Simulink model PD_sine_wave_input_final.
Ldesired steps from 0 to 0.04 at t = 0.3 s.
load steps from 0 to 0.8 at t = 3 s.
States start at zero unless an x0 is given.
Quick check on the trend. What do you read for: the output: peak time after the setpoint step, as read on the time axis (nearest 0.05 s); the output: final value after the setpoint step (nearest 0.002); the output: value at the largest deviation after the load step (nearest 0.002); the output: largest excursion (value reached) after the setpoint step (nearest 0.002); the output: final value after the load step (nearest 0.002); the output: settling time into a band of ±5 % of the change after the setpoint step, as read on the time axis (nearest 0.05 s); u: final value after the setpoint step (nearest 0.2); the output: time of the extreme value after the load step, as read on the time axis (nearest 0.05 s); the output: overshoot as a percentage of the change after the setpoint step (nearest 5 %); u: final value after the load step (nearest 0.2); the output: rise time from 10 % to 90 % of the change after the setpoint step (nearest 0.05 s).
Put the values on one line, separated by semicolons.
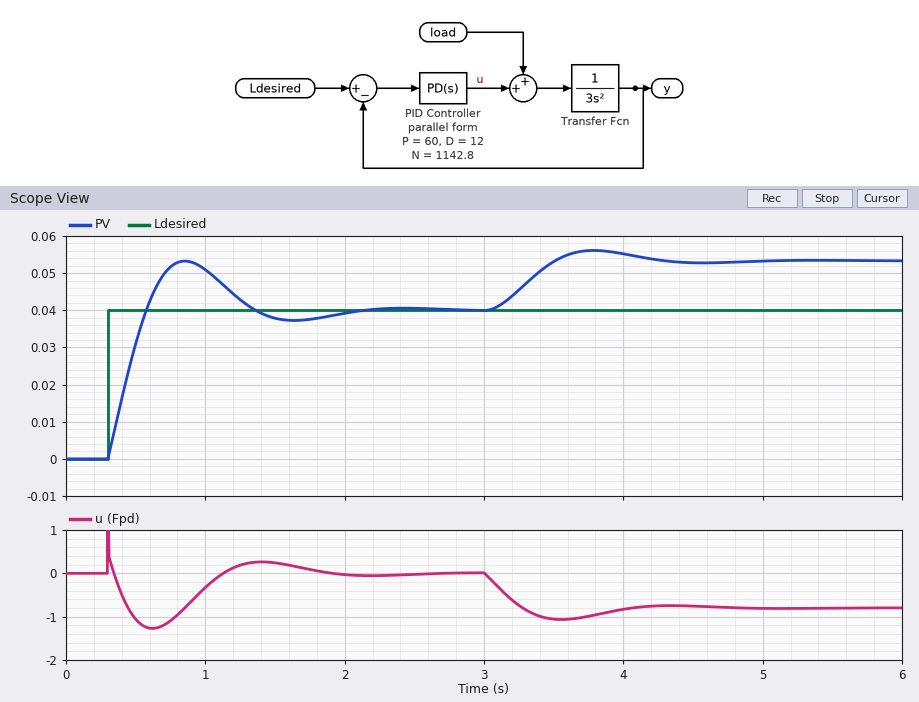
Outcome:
0.85 s; 0.040; 0.056; 0.054; 0.054; 1.85 s; 0.0; 3.80 s; 35 %; -0.8; 0.20 s
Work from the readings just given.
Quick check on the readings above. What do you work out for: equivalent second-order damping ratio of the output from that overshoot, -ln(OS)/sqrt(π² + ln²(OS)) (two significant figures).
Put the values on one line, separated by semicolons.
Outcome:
0.32
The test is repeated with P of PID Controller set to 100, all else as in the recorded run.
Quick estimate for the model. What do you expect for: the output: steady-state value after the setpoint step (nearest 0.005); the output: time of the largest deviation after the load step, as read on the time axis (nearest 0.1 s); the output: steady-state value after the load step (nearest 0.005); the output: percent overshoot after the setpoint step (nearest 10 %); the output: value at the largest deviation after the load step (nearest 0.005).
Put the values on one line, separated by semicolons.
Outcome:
0.040; 3.6 s; 0.050; 40 %; 0.050
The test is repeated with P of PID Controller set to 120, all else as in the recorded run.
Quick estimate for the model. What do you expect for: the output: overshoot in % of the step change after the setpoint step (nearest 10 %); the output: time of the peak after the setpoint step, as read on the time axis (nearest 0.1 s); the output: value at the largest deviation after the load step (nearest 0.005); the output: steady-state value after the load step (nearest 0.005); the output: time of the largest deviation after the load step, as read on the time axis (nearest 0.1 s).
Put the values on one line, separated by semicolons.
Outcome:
40 %; 0.7 s; 0.050; 0.045; 3.5 s
